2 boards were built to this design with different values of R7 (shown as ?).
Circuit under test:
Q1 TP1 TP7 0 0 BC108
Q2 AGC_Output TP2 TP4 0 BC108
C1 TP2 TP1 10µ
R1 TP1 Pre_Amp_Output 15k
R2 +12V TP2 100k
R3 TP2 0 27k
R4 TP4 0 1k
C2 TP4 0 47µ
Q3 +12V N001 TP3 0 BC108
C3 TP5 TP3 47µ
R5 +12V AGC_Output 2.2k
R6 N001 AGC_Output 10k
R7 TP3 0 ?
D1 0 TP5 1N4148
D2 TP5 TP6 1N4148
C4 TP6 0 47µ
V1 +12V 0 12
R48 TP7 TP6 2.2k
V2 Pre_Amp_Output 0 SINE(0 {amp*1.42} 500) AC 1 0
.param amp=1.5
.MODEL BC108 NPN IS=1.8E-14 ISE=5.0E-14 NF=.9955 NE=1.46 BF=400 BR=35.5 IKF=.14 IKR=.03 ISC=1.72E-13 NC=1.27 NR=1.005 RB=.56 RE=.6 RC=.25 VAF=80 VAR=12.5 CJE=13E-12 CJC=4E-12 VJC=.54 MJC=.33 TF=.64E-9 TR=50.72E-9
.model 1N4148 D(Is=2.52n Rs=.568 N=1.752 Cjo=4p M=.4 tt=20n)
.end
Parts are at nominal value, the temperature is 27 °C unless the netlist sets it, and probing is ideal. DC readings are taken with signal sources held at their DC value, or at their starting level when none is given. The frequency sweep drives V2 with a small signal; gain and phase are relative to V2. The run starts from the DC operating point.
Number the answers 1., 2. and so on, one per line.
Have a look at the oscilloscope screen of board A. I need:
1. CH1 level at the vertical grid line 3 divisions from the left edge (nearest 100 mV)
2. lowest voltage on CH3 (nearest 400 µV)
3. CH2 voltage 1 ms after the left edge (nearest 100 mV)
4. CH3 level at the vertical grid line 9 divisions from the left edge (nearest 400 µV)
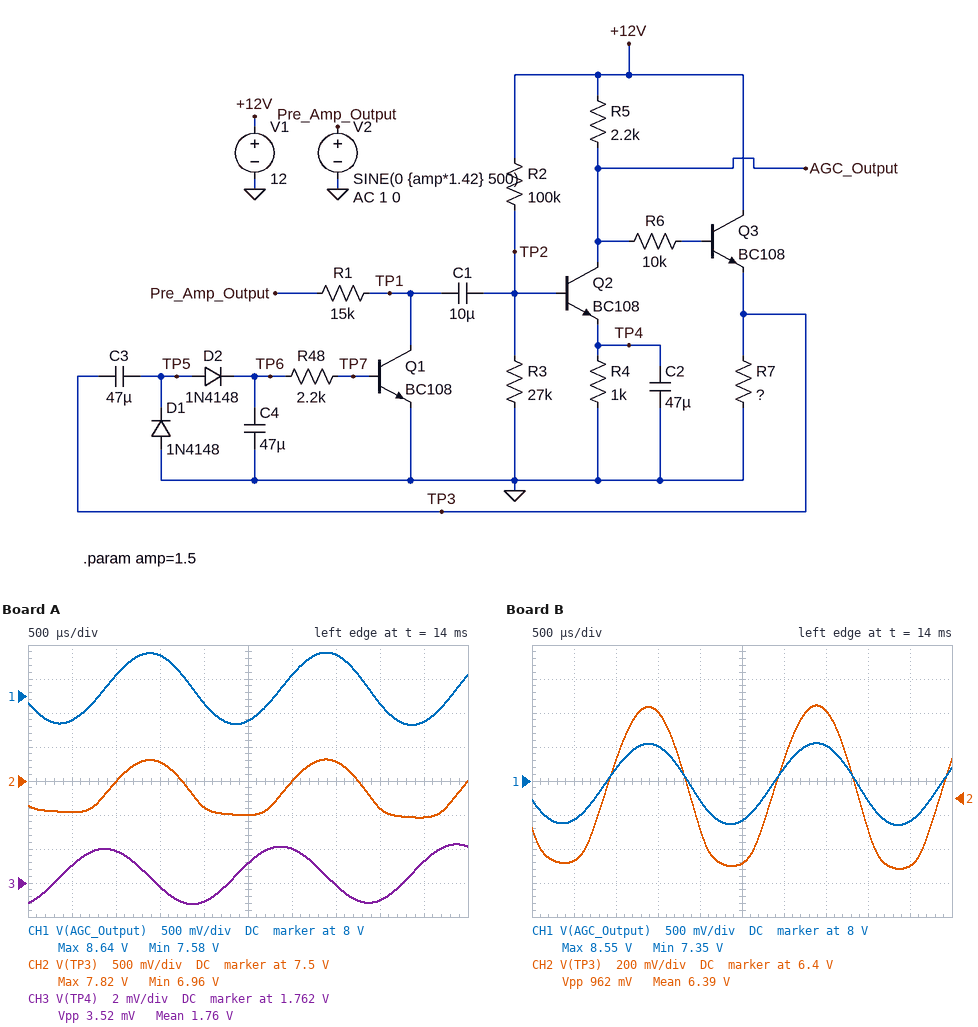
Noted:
1. 8.6 V
2. 1.7608 V
3. 7.5 V
4. 1.7632 V
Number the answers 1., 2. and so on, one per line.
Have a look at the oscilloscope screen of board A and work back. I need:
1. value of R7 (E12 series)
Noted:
1. 1.8 kΩ
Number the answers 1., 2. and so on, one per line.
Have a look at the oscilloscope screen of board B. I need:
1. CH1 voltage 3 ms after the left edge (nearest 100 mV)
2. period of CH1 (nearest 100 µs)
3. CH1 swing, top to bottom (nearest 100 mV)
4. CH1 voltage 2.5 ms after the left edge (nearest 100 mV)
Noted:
1. 8.2 V
2. 2.0 ms
3. 1.2 V
4. 7.4 V
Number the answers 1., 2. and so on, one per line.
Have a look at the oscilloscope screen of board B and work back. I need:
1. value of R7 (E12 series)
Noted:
1. 270 Ω
